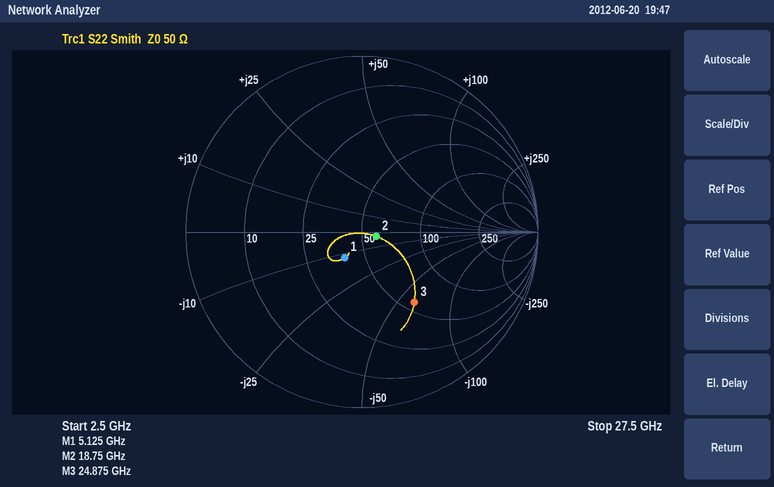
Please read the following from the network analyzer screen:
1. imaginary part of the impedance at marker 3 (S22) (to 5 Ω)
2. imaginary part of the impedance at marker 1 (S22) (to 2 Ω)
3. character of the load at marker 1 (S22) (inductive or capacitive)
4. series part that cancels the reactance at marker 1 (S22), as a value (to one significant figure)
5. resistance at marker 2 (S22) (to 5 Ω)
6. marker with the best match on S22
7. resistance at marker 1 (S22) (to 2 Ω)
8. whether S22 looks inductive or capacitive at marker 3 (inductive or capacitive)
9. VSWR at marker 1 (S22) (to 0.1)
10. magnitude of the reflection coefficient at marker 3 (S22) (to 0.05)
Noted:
-60 Ω
-12 Ω
capacitive
400 pH
60 Ω
marker 2
40 Ω
capacitive
1.4
0.50
